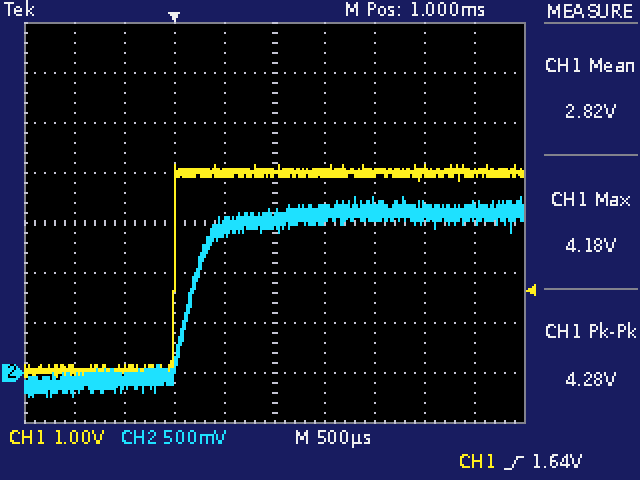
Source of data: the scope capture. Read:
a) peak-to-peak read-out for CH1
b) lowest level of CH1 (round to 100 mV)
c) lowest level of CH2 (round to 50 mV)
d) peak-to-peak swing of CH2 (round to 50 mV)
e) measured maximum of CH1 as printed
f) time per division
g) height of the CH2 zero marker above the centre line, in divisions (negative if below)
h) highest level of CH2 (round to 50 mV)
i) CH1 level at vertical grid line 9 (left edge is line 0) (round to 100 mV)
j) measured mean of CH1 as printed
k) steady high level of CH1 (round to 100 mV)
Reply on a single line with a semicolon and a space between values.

4.28 V; -100 mV; -250 mV; 2.00 V; 4.18 V; 500 µs; -3.0 div; 1.75 V; 4.0 V; 2.82 V; 4.0 V
